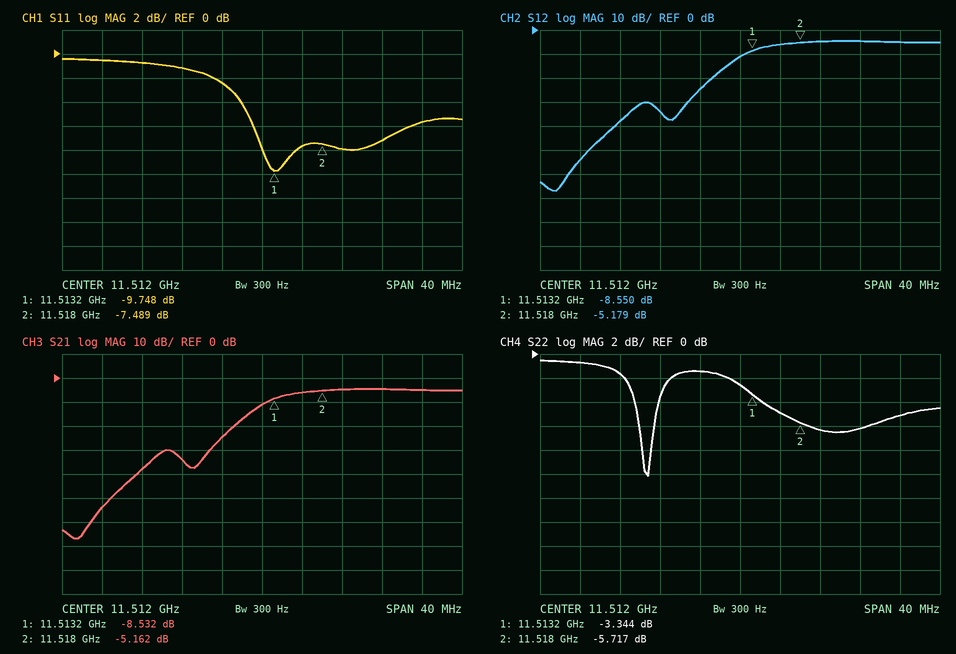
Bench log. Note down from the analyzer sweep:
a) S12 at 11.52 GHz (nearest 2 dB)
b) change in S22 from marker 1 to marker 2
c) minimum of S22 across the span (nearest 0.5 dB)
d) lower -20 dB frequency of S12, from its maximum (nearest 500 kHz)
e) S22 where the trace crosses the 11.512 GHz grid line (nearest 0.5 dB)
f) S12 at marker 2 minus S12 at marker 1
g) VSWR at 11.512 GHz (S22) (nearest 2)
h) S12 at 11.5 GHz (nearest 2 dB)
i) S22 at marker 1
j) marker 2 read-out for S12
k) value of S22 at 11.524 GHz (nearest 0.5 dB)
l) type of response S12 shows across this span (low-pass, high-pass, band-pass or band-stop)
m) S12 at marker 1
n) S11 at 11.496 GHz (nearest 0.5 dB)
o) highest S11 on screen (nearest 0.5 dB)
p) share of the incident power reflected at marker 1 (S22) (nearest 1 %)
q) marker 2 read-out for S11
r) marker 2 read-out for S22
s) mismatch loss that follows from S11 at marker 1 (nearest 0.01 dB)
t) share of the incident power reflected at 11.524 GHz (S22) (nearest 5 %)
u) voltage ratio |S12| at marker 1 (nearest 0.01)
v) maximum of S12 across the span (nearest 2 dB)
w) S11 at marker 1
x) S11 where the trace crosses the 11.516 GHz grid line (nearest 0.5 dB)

-4 dB
-2.373 dB
-10.0 dB
11.5080 GHz
-2.5 dB
3.371 dB
6
-38 dB
-3.344 dB
-5.179 dB
-6.0 dB
high-pass
-8.550 dB
-0.5 dB
-0.5 dB
46 %
-7.489 dB
-5.717 dB
0.49 dB
25 %
0.37
-4 dB
-9.748 dB
-7.5 dB
